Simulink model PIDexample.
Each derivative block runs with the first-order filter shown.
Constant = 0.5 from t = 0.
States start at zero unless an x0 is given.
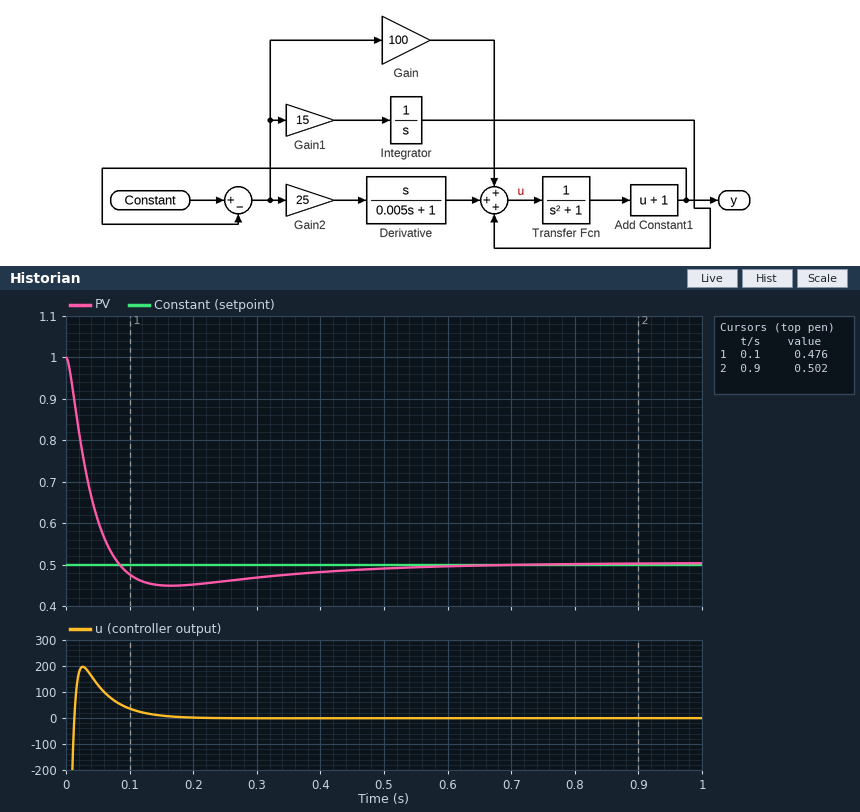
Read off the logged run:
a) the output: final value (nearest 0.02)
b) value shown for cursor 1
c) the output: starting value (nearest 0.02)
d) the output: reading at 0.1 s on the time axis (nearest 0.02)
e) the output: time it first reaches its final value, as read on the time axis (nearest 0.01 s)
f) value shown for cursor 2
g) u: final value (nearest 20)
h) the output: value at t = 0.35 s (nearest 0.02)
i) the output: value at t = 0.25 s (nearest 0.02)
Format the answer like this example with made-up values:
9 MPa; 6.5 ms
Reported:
0.50; 0.476; 1.00; 0.48; 0.08 s; 0.502; 0; 0.48; 0.46
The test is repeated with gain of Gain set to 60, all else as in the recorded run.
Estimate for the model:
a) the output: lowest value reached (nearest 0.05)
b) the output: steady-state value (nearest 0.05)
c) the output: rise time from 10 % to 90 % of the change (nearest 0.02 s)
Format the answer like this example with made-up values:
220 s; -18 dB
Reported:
0.45; 0.50; 0.06 s
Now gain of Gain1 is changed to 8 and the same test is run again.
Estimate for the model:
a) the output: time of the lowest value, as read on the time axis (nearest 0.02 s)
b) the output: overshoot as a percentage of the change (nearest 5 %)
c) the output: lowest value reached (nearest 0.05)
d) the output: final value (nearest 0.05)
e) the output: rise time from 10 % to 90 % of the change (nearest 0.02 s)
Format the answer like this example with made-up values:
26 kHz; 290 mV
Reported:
0.16 s; 10 %; 0.45; 0.50; 0.06 s
